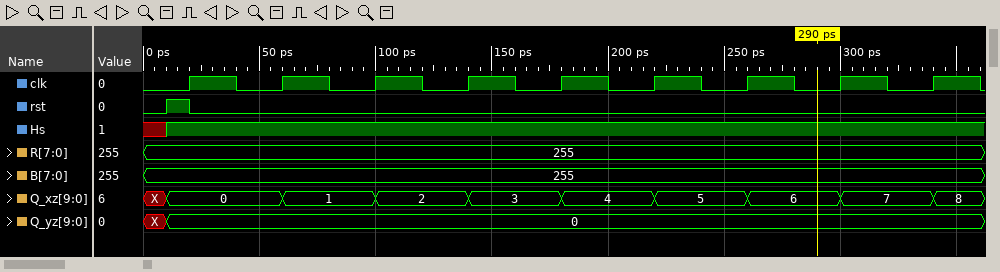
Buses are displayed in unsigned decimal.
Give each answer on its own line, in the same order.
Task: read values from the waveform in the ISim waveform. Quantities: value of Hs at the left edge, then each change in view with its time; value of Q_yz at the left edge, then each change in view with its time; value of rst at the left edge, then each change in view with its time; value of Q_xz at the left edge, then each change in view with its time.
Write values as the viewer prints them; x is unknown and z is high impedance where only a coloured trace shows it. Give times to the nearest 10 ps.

x, 1 at 10 ps
X, 0 at 10 ps
0, 1 at 10 ps, 0 at 20 ps
X, 0 at 10 ps, 1 at 60 ps, 2 at 100 ps, 3 at 140 ps, 4 at 180 ps, 5 at 220 ps, 6 at 260 ps, 7 at 300 ps, 8 at 340 ps
